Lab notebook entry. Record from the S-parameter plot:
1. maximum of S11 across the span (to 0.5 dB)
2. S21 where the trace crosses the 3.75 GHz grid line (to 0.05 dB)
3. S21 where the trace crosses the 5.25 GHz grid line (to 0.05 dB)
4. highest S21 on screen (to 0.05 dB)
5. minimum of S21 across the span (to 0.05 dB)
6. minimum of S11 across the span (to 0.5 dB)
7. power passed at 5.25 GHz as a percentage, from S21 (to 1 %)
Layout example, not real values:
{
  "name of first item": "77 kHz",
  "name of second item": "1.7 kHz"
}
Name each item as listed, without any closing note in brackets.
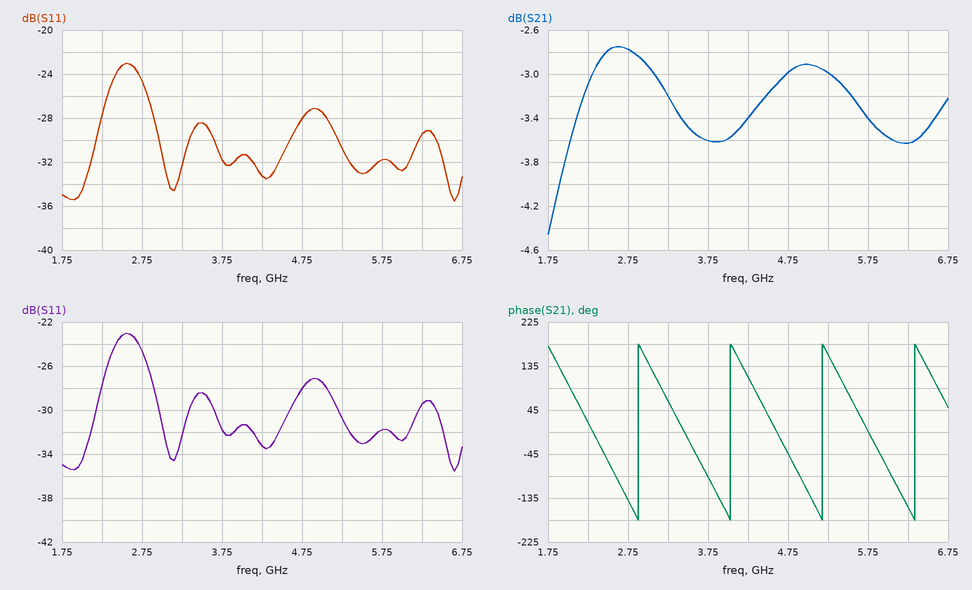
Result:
{
  "maximum of S11 across the span": "-23.0 dB",
  "S21 where the trace crosses the 3.75 GHz grid line": "-3.60 dB",
  "S21 where the trace crosses the 5.25 GHz grid line": "-3.00 dB",
  "highest S21 on screen": "-2.75 dB",
  "minimum of S21 across the span": "-4.45 dB",
  "minimum of S11 across the span": "-35.5 dB",
  "power passed at 5.25 GHz as a percentage, from S21": "50 %"
}
